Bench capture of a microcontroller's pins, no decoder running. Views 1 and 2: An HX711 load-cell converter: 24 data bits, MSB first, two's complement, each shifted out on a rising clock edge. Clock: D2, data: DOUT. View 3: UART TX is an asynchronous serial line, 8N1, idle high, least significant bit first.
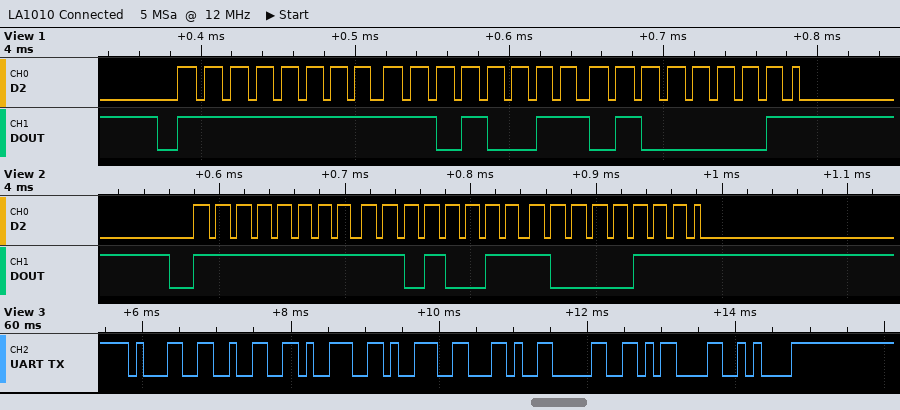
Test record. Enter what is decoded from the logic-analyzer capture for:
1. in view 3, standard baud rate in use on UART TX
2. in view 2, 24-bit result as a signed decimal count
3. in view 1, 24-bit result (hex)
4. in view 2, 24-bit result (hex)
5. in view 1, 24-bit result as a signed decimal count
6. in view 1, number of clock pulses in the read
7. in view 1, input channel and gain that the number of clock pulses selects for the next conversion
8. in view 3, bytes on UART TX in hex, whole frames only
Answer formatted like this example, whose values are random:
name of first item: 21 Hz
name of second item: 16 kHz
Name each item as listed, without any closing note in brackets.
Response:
in view 3, standard baud rate in use on UART TX: 9600 baud
in view 2, 24-bit result as a signed decimal count: -11385
in view 1, 24-bit result: 0xFFD341
in view 2, 24-bit result: 0xFFD387
in view 1, 24-bit result as a signed decimal count: -11455
in view 1, number of clock pulses in the read: 25
in view 1, input channel and gain that the number of clock pulses selects for the next conversion: channel A, gain 128
in view 3, bytes on UART TX in hex, whole frames only: 31 32 39 39 2C 30 0D 0A
